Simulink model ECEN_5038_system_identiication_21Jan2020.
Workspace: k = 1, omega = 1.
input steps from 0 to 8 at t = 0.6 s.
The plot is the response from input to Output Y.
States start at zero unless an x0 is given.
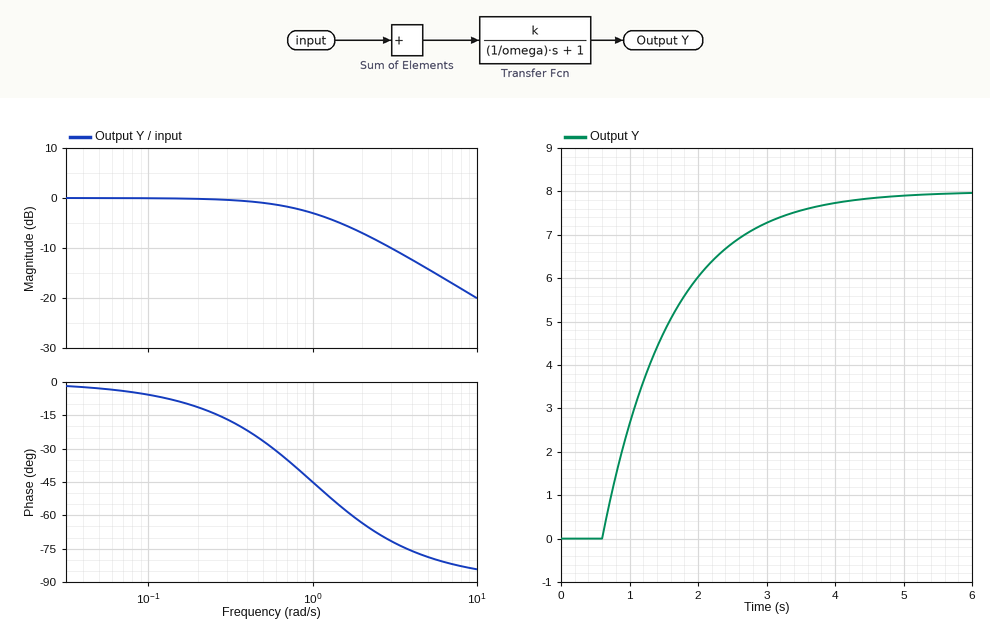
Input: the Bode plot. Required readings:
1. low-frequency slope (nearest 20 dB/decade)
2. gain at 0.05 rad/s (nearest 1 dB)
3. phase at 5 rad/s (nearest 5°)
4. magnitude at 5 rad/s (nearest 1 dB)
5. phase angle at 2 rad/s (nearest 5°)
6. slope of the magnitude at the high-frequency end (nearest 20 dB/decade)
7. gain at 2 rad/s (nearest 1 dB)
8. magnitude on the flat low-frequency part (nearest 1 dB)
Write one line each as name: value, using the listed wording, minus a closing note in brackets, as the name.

low-frequency slope: 0 dB/decade
gain at 0.05 rad/s: 0 dB
phase at 5 rad/s: -80°
magnitude at 5 rad/s: -14 dB
phase angle at 2 rad/s: -65°
slope of the magnitude at the high-frequency end: -20 dB/decade
gain at 2 rad/s: -7 dB
magnitude on the flat low-frequency part: 0 dB
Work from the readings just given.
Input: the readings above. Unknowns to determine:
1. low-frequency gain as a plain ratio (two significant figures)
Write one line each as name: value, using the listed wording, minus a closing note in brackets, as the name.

low-frequency gain as a plain ratio: 1.0
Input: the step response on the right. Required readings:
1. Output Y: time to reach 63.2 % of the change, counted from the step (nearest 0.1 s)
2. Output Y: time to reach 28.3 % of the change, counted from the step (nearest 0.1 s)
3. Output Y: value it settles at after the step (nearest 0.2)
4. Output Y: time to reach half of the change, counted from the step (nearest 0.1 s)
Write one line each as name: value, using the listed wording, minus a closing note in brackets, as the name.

Output Y: time to reach 63.2 % of the change, counted from the step: 1.0 s
Output Y: time to reach 28.3 % of the change, counted from the step: 0.3 s
Output Y: value it settles at after the step: 8.0
Output Y: time to reach half of the change, counted from the step: 0.7 s
